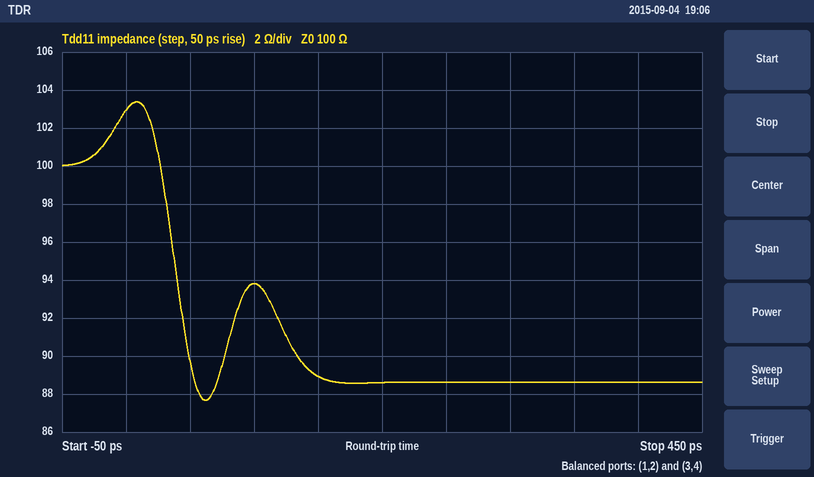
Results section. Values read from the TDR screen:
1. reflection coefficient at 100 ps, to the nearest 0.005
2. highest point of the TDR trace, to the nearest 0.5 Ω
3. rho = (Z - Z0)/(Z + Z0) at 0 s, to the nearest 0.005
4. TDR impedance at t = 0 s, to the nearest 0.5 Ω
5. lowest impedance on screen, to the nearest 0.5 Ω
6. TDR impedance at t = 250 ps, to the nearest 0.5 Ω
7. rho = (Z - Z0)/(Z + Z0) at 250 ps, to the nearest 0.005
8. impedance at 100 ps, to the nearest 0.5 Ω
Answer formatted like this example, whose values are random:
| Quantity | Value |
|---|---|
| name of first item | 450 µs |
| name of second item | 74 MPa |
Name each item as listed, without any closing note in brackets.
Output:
| Quantity | Value |
|---|---|
| reflection coefficient at 100 ps, to the nearest 0.005 | -0.030 |
| highest point of the TDR trace, to the nearest 0.5 Ω | 103.5 Ω |
| rho = (Z - Z0)/(Z + Z0) at 0 s, to the nearest 0.005 | +0.015 |
| TDR impedance at t = 0 s, to the nearest 0.5 Ω | 103.0 Ω |
| lowest impedance on screen, to the nearest 0.5 Ω | 87.5 Ω |
| TDR impedance at t = 250 ps, to the nearest 0.5 Ω | 88.5 Ω |
| rho = (Z - Z0)/(Z + Z0) at 250 ps, to the nearest 0.005 | -0.060 |
| impedance at 100 ps, to the nearest 0.5 Ω | 94.0 Ω |
